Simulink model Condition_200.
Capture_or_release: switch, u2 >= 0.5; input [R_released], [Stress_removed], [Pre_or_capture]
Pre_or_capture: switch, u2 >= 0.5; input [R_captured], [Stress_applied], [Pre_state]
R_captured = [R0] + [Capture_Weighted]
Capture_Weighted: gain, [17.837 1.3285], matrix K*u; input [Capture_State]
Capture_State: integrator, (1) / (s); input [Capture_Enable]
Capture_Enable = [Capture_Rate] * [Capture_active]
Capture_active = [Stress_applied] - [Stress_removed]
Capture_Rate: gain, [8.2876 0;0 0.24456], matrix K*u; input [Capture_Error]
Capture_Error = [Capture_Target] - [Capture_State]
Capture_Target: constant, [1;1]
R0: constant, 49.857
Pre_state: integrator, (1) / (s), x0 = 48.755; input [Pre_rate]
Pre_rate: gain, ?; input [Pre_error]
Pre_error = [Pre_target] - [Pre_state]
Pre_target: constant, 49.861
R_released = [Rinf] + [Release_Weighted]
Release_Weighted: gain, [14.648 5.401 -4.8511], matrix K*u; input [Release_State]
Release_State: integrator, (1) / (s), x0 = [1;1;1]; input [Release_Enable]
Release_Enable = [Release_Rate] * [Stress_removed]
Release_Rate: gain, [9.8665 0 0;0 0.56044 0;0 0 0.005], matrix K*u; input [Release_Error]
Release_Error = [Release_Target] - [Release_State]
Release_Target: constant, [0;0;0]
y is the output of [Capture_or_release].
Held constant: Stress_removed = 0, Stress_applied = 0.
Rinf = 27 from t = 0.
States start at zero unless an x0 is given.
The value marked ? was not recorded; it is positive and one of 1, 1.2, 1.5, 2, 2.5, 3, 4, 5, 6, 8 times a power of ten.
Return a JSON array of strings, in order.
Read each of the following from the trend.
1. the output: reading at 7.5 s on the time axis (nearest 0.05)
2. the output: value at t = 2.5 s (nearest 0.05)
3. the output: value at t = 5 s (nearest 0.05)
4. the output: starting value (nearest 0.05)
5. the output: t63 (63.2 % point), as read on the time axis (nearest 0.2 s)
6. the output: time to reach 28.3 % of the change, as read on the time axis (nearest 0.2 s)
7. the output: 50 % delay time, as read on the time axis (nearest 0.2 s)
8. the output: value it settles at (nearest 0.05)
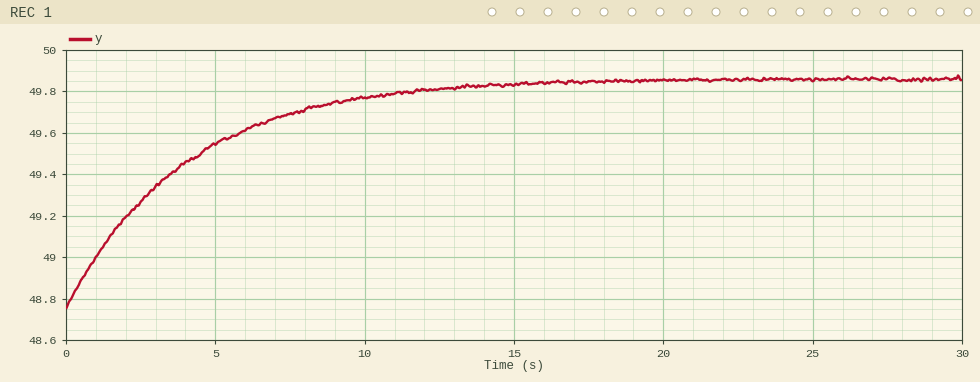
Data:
["49.70", "49.25", "49.55", "48.75", "4.0 s", "1.4 s", "2.8 s", "49.85"]
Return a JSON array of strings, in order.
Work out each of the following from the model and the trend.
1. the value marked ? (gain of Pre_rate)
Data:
["0.25"]
